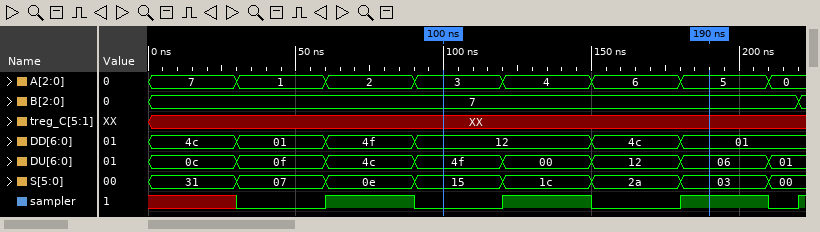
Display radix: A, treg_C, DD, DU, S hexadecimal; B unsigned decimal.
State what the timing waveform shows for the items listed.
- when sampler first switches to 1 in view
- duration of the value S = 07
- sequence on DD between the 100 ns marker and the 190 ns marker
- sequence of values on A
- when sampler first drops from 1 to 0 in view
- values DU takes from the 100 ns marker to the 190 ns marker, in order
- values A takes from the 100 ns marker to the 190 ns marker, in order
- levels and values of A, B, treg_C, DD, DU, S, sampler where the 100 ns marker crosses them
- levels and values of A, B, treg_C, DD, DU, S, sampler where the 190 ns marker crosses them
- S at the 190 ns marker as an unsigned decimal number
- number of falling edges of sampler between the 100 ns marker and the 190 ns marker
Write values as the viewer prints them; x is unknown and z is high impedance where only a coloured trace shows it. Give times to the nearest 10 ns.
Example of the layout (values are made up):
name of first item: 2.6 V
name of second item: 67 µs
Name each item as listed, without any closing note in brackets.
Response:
when sampler first switches to 1 in view: 60 ns
duration of the value S = 07: 30 ns
sequence on DD between the 100 ns marker and the 190 ns marker: 12, 4c, 01
sequence of values on A: 7, 1, 2, 3, 4, 6, 5, 0
when sampler first drops from 1 to 0 in view: 90 ns
values DU takes from the 100 ns marker to the 190 ns marker, in order: 4f, 00, 12, 06
values A takes from the 100 ns marker to the 190 ns marker, in order: 3, 4, 6, 5
levels and values of A, B, treg_C, DD, DU, S, sampler where the 100 ns marker crosses them: A=3, B=7, treg_C=XX, DD=12, DU=4f, S=15, sampler=0
levels and values of A, B, treg_C, DD, DU, S, sampler where the 190 ns marker crosses them: A=5, B=7, treg_C=XX, DD=01, DU=06, S=03, sampler=1
S at the 190 ns marker as an unsigned decimal number: 3
number of falling edges of sampler between the 100 ns marker and the 190 ns marker: 1
